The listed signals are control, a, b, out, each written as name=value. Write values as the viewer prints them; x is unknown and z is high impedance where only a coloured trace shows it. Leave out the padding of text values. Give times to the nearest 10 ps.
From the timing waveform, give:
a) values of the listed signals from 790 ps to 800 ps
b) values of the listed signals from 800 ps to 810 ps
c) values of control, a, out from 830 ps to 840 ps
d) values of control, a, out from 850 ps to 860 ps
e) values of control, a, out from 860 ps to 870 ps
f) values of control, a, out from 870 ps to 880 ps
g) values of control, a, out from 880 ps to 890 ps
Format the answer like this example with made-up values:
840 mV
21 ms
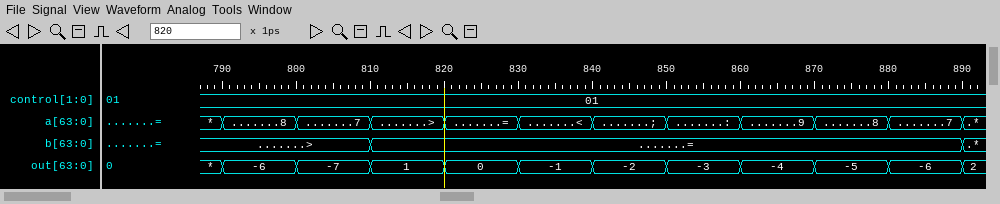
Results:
control=01, a=8, b=>, out=-6
control=01, a=7, b=>, out=-7
control=01, a=<, out=-1
control=01, a=:, out=-3
control=01, a=9, out=-4
control=01, a=8, out=-5
control=01, a=7, out=-6
